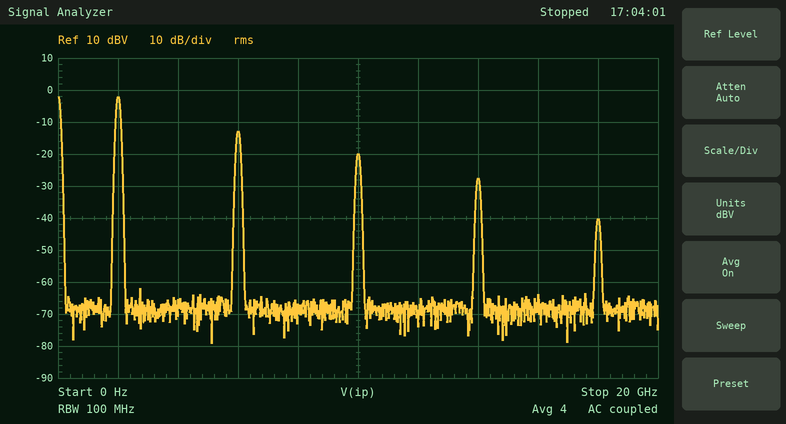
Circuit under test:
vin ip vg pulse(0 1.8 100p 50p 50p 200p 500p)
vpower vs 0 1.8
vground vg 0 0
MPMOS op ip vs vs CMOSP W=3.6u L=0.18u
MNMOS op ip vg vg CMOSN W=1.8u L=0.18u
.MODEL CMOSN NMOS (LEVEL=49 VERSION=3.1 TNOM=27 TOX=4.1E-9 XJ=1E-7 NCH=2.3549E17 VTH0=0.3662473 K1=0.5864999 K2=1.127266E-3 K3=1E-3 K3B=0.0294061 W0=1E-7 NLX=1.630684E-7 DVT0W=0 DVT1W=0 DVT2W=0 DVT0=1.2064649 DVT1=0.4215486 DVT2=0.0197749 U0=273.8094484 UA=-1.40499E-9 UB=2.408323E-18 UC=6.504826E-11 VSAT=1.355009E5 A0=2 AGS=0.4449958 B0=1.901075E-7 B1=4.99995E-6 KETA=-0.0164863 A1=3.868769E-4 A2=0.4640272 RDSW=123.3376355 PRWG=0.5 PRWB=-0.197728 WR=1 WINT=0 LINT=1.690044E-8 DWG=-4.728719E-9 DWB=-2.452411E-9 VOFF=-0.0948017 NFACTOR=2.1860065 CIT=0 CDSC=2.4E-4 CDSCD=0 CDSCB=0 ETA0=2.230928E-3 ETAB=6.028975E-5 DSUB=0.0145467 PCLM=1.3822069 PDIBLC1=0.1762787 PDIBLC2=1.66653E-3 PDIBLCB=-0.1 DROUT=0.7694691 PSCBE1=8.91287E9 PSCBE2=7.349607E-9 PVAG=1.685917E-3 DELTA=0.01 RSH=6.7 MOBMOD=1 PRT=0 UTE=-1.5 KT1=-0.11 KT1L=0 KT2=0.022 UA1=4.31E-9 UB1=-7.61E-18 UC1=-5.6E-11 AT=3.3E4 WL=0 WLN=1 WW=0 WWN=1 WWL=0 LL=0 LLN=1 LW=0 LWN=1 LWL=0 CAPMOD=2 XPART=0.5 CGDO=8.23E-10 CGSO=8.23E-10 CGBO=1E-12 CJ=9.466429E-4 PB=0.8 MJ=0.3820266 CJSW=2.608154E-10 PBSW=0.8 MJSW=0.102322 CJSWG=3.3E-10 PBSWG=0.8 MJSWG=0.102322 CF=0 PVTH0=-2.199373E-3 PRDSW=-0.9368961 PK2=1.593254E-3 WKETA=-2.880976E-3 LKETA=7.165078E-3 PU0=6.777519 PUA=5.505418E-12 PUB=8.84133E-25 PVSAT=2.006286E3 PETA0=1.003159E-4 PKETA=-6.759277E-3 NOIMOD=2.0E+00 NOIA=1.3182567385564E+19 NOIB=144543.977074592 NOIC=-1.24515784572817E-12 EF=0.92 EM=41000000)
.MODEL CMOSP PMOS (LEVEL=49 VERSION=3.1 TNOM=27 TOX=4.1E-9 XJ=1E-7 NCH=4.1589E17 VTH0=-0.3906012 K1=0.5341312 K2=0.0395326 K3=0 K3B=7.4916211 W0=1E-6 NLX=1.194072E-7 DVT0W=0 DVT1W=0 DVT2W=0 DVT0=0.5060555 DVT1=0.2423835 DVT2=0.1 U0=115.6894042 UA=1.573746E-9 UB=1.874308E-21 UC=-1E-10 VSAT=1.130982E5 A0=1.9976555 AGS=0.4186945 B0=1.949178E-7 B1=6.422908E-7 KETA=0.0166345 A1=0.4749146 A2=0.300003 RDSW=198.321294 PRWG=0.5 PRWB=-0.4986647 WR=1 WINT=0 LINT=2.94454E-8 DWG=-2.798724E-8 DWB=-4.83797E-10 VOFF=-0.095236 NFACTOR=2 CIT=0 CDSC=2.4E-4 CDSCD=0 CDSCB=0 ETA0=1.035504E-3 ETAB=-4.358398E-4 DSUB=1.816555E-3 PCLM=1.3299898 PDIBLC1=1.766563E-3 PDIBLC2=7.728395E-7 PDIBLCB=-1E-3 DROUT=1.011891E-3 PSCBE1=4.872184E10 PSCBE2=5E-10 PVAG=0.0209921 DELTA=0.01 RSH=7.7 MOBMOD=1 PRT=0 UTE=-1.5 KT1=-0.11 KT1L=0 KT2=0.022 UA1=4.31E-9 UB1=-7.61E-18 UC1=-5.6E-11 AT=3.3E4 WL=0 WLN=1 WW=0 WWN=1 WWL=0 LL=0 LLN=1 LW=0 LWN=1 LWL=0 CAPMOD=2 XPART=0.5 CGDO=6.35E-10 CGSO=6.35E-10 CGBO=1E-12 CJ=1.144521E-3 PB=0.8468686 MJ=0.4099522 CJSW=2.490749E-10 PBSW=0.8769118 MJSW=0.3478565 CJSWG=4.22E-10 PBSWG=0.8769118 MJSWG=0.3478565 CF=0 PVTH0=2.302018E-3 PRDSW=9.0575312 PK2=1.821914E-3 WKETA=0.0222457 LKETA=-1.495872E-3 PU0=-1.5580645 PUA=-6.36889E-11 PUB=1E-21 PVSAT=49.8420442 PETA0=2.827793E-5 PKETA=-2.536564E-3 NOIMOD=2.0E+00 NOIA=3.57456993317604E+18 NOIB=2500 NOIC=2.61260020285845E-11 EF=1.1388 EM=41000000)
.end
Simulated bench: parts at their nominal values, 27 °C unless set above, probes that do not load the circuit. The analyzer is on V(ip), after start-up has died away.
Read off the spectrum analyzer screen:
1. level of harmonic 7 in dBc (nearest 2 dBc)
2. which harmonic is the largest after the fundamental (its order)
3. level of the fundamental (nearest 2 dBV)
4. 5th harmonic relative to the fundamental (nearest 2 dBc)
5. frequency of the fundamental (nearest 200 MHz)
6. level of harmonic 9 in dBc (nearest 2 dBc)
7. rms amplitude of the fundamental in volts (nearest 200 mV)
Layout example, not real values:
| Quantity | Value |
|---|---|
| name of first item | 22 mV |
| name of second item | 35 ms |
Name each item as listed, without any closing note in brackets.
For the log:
| Quantity | Value |
|---|---|
| level of harmonic 7 in dBc | -26 dBc |
| which harmonic is the largest after the fundamental | 3 |
| level of the fundamental | -2 dBV |
| 5th harmonic relative to the fundamental | -18 dBc |
| frequency of the fundamental | 2.0 GHz |
| level of harmonic 9 in dBc | -38 dBc |
| rms amplitude of the fundamental in volts | 800 mV |
